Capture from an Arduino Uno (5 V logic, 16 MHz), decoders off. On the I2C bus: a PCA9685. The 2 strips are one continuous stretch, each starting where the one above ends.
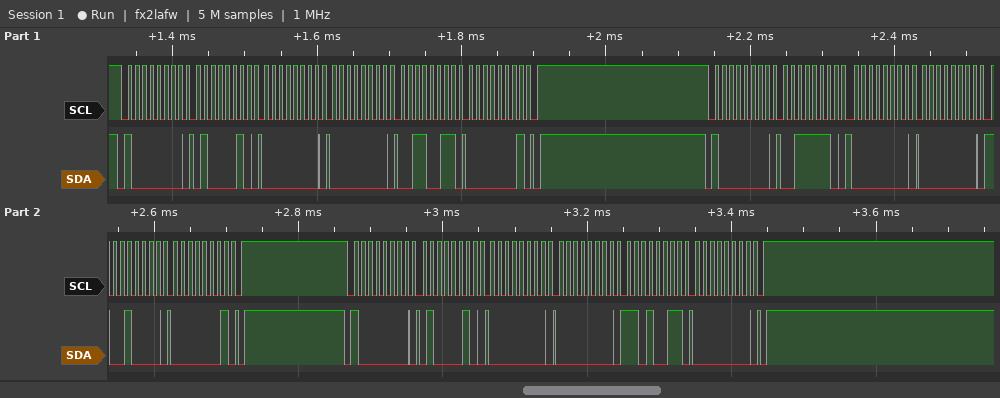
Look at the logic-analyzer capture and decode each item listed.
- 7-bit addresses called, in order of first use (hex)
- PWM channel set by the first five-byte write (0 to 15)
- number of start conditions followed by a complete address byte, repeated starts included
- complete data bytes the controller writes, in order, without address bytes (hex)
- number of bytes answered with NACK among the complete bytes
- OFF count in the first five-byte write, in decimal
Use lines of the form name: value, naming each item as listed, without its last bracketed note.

7-bit addresses called, in order of first use: 0x40
PWM channel set by the first five-byte write: 15
number of start conditions followed by a complete address byte, repeated starts included: 3
complete data bytes the controller writes, in order, without address bytes: 42 00 00 33 01 3E 00 00 90 01 42 00 00 D3 00
number of bytes answered with NACK among the complete bytes: 0
OFF count in the first five-byte write, in decimal: 307
